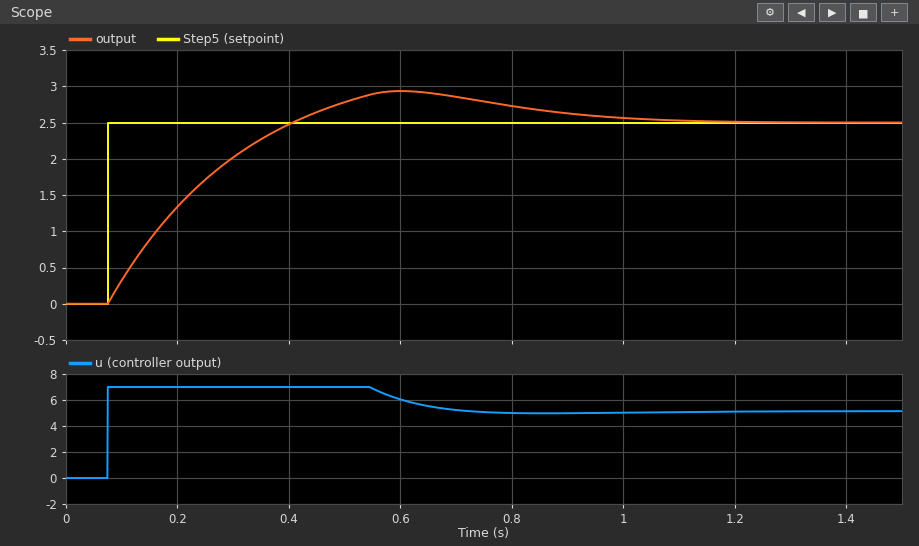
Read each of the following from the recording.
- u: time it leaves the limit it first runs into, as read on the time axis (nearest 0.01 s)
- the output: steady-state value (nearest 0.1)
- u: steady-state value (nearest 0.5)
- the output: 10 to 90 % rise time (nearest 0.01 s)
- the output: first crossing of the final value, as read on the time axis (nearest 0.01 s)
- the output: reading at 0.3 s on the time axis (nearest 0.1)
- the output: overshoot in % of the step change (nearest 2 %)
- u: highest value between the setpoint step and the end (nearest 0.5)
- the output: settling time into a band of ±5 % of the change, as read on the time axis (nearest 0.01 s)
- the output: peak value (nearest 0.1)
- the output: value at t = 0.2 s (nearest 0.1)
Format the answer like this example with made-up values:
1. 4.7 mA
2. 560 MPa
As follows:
1. 0.55 s
2. 2.5
3. 5.0
4. 0.25 s
5. 0.41 s
6. 2.0
7. 18 %
8. 7.0
9. 0.90 s
10. 2.9
11. 1.3
